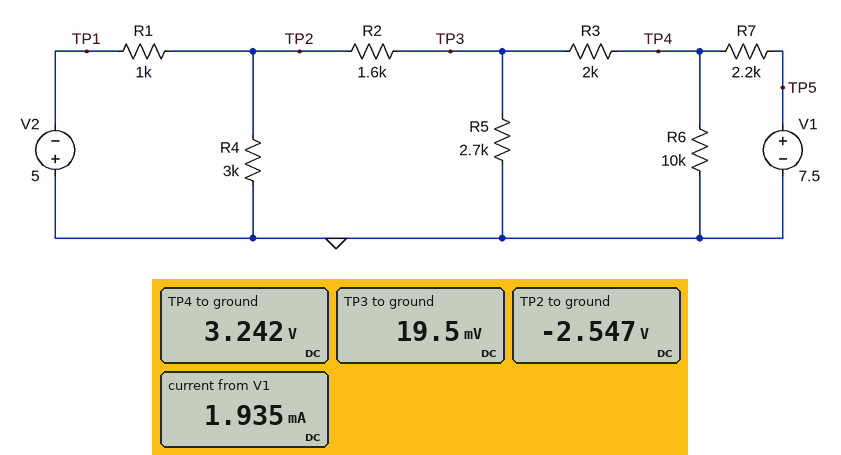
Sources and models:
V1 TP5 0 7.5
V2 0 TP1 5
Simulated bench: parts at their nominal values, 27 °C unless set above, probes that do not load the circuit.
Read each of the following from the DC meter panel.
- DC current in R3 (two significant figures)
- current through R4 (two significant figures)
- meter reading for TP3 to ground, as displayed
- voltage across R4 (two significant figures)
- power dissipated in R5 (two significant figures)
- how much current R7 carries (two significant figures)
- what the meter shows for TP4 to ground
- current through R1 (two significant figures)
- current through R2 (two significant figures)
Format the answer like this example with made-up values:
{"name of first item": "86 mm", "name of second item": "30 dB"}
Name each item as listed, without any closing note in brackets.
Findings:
{"DC current in R3": "1.6 mA", "current through R4": "850 µA", "meter reading for TP3 to ground, as displayed": "19.5 mV", "voltage across R4": "2.5 V", "power dissipated in R5": "140 nW", "how much current R7 carries": "1.9 mA", "what the meter shows for TP4 to ground": "3.242 V", "current through R1": "2.5 mA", "current through R2": "1.6 mA"}
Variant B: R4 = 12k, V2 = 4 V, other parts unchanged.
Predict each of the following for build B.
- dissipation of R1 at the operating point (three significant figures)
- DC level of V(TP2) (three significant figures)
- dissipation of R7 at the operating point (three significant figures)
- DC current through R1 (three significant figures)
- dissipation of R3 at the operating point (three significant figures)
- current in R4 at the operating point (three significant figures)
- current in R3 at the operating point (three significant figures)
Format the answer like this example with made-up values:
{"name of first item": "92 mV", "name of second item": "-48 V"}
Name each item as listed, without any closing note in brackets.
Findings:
{"dissipation of R1 at the operating point": "2.93 mW", "DC level of V(TP2)": "-2.29 V", "dissipation of R7 at the operating point": "8.01 mW", "DC current through R1": "1.71 mA", "dissipation of R3 at the operating point": "4.98 mW", "current in R4 at the operating point": "191 µA", "current in R3 at the operating point": "1.58 mA"}
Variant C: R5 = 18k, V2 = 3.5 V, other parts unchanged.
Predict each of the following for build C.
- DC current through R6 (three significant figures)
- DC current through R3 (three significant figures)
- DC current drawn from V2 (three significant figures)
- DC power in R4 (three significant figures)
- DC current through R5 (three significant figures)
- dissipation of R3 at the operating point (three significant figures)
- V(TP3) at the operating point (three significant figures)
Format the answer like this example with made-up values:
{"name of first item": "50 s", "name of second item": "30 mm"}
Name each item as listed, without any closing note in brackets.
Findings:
{"DC current through R6": "355 µA", "DC current through R3": "1.44 mA", "DC current drawn from V2": "1.93 mA", "DC power in R4": "825 µW", "DC current through R5": "37.3 µA", "dissipation of R3 at the operating point": "4.15 mW", "V(TP3) at the operating point": "671 mV"}
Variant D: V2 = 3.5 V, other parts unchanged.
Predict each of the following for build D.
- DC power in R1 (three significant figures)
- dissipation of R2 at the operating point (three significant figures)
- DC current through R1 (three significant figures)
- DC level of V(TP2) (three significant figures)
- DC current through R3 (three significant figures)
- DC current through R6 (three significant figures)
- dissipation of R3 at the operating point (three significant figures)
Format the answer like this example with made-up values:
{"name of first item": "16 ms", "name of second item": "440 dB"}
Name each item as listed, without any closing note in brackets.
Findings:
{"DC power in R1": "3.47 mW", "dissipation of R2 at the operating point": "2.78 mW", "DC current through R1": "1.86 mA", "DC level of V(TP2)": "-1.64 V", "DC current through R3": "1.49 mA", "DC current through R6": "346 µA", "dissipation of R3 at the operating point": "4.45 mW"}
